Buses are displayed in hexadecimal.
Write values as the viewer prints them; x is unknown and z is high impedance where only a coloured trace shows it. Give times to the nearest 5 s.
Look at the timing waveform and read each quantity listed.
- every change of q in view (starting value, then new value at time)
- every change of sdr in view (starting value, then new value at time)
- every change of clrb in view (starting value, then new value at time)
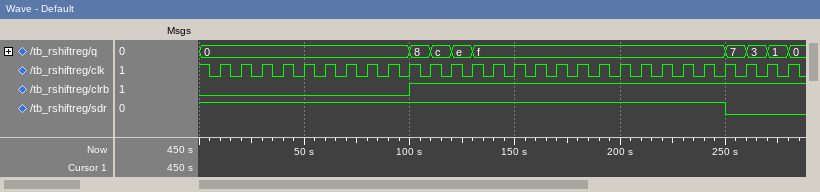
0, 8 at 100 s, c at 110 s, e at 120 s, f at 130 s, 7 at 250 s, 3 at 260 s, 1 at 270 s, 0 at 280 s
1, 0 at 250 s
0, 1 at 100 s
